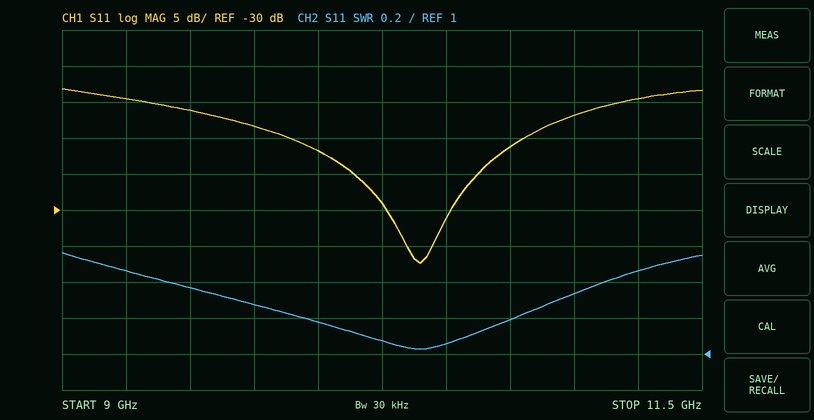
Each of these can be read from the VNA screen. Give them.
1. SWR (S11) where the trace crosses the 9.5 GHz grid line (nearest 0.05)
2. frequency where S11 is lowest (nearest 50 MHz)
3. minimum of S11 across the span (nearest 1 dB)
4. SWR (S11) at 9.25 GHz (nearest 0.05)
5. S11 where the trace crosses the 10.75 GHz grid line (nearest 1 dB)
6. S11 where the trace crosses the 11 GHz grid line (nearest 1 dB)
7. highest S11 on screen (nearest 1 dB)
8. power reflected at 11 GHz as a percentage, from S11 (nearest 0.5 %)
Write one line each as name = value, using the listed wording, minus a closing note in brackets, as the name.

SWR (S11) where the trace crosses the 9.5 GHz grid line = 1.35
frequency where S11 is lowest = 10.40 GHz
minimum of S11 across the span = -37 dB
SWR (S11) at 9.25 GHz = 1.45
S11 where the trace crosses the 10.75 GHz grid line = -21 dB
S11 where the trace crosses the 11 GHz grid line = -17 dB
highest S11 on screen = -13 dB
power reflected at 11 GHz as a percentage, from S11 = 2.0 %
